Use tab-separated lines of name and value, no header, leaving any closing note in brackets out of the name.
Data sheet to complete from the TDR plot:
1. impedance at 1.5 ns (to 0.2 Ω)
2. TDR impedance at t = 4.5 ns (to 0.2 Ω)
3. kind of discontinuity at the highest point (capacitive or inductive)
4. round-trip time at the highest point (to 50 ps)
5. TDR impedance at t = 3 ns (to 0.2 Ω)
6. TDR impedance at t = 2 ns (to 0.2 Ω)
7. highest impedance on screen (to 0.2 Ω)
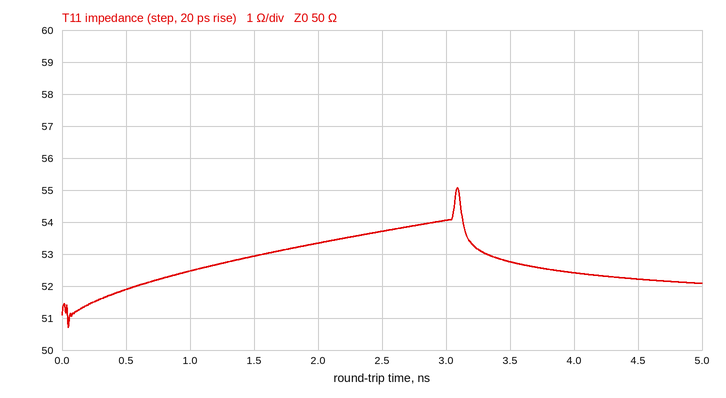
impedance at 1.5 ns	53.0 Ω
TDR impedance at t = 4.5 ns	52.2 Ω
kind of discontinuity at the highest point	inductive
round-trip time at the highest point	3.10 ns
TDR impedance at t = 3 ns	54.0 Ω
TDR impedance at t = 2 ns	53.4 Ω
highest impedance on screen	55.0 Ω
